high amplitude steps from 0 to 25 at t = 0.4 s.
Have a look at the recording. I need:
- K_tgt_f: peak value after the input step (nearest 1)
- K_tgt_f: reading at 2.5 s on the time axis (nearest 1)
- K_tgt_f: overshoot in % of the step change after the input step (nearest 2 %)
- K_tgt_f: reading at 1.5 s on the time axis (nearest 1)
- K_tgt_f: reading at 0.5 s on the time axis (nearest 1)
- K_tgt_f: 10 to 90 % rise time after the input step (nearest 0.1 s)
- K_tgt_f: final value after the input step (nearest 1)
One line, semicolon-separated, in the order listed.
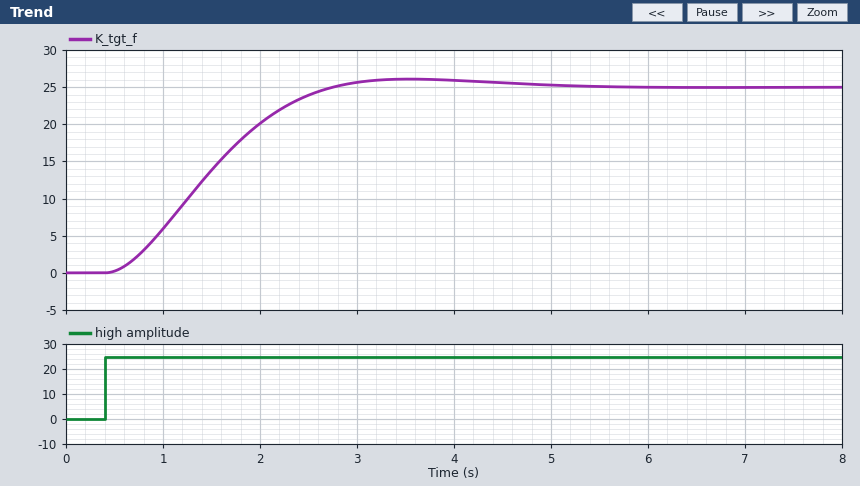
26; 24; 4 %; 14; 0; 1.5 s; 25
